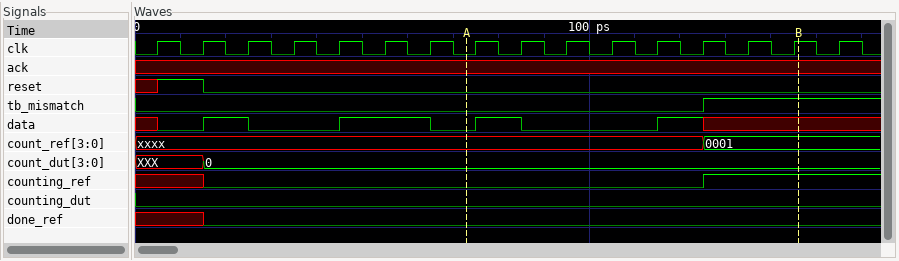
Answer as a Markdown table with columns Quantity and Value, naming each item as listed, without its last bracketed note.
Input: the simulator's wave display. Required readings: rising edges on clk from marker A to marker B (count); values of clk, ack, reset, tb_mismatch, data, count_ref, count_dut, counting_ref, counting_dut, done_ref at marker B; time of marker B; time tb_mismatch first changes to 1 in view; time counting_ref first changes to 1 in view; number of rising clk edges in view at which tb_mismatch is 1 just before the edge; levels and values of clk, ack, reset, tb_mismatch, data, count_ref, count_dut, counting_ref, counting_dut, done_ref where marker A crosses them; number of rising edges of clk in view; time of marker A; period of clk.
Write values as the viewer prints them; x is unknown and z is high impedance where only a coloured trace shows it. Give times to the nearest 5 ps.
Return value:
| Quantity | Value |
|---|---|
| rising edges on clk from marker A to marker B | 8 |
| values of clk, ack, reset, tb_mismatch, data, count_ref, count_dut, counting_ref, counting_dut, done_ref at marker B | clk=1, ack=x, reset=0, tb_mismatch=1, data=x, count_ref=0001, count_dut=0, counting_ref=1, counting_dut=0, done_ref=0 |
| time of marker B | 145 ps |
| time tb_mismatch first changes to 1 in view | 125 ps |
| time counting_ref first changes to 1 in view | 125 ps |
| number of rising clk edges in view at which tb_mismatch is 1 just before the edge | 3 |
| levels and values of clk, ack, reset, tb_mismatch, data, count_ref, count_dut, counting_ref, counting_dut, done_ref where marker A crosses them | clk=0, ack=x, reset=0, tb_mismatch=0, data=0, count_ref=xxxx, count_dut=0, counting_ref=0, counting_dut=0, done_ref=0 |
| number of rising edges of clk in view | 16 |
| time of marker A | 75 ps |
| period of clk | 10 ps |
